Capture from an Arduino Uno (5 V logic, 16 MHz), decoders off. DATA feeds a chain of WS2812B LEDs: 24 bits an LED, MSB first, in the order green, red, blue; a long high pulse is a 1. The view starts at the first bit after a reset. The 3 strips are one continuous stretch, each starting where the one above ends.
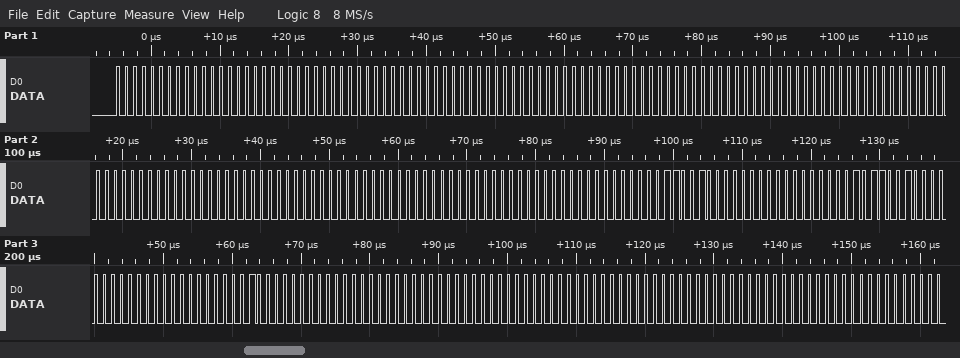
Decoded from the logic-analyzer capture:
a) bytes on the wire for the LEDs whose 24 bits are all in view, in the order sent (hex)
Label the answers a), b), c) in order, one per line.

a) 00 00 00 00 00 00 00 00 00 00 00 00 00 00 00 00 00 00 00 00 19 00 00 59 00 00 02 00 00 00 00 00 00 00 00 00
